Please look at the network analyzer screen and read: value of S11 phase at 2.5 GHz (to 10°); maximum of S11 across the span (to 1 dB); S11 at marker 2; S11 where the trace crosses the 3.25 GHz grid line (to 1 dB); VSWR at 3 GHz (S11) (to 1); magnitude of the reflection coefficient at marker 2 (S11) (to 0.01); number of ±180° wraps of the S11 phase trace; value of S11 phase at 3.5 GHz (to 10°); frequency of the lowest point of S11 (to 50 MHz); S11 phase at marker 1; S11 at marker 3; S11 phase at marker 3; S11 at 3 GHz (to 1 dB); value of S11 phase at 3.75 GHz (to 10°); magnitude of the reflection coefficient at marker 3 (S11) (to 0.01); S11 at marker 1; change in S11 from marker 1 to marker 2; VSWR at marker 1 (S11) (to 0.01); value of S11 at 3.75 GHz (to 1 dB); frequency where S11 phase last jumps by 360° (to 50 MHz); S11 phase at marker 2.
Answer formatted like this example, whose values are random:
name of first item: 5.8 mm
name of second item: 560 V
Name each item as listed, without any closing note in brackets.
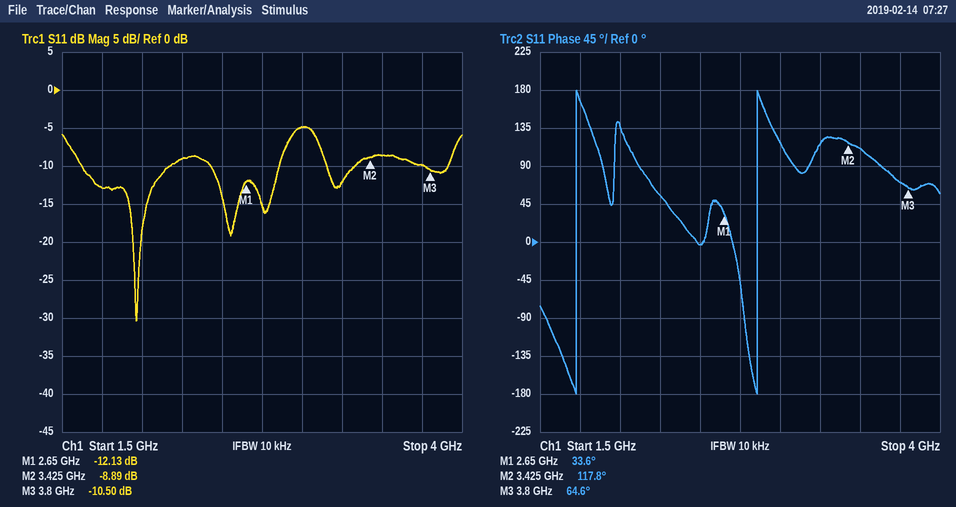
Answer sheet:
value of S11 phase at 2.5 GHz: 0°
maximum of S11 across the span: -5 dB
S11 at marker 2: -8.89 dB
S11 where the trace crosses the 3.25 GHz grid line: -12 dB
VSWR at 3 GHz (S11): 4
magnitude of the reflection coefficient at marker 2 (S11): 0.36
number of ±180° wraps of the S11 phase trace: 2
value of S11 phase at 3.5 GHz: 110°
frequency of the lowest point of S11: 1.95 GHz
S11 phase at marker 1: 33.6°
S11 at marker 3: -10.50 dB
S11 phase at marker 3: 64.6°
S11 at 3 GHz: -5 dB
value of S11 phase at 3.75 GHz: 70°
magnitude of the reflection coefficient at marker 3 (S11): 0.30
S11 at marker 1: -12.13 dB
change in S11 from marker 1 to marker 2: 3.24 dB
VSWR at marker 1 (S11): 1.66
value of S11 at 3.75 GHz: -10 dB
frequency where S11 phase last jumps by 360°: 2.85 GHz
S11 phase at marker 2: 117.8°
